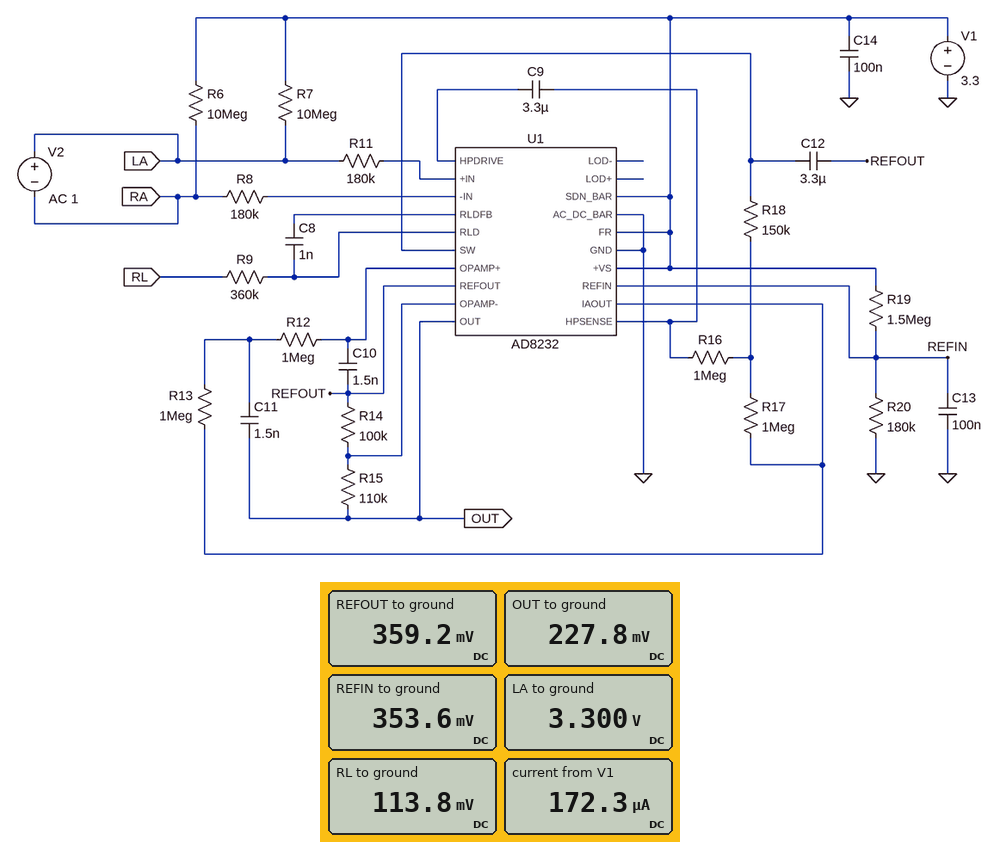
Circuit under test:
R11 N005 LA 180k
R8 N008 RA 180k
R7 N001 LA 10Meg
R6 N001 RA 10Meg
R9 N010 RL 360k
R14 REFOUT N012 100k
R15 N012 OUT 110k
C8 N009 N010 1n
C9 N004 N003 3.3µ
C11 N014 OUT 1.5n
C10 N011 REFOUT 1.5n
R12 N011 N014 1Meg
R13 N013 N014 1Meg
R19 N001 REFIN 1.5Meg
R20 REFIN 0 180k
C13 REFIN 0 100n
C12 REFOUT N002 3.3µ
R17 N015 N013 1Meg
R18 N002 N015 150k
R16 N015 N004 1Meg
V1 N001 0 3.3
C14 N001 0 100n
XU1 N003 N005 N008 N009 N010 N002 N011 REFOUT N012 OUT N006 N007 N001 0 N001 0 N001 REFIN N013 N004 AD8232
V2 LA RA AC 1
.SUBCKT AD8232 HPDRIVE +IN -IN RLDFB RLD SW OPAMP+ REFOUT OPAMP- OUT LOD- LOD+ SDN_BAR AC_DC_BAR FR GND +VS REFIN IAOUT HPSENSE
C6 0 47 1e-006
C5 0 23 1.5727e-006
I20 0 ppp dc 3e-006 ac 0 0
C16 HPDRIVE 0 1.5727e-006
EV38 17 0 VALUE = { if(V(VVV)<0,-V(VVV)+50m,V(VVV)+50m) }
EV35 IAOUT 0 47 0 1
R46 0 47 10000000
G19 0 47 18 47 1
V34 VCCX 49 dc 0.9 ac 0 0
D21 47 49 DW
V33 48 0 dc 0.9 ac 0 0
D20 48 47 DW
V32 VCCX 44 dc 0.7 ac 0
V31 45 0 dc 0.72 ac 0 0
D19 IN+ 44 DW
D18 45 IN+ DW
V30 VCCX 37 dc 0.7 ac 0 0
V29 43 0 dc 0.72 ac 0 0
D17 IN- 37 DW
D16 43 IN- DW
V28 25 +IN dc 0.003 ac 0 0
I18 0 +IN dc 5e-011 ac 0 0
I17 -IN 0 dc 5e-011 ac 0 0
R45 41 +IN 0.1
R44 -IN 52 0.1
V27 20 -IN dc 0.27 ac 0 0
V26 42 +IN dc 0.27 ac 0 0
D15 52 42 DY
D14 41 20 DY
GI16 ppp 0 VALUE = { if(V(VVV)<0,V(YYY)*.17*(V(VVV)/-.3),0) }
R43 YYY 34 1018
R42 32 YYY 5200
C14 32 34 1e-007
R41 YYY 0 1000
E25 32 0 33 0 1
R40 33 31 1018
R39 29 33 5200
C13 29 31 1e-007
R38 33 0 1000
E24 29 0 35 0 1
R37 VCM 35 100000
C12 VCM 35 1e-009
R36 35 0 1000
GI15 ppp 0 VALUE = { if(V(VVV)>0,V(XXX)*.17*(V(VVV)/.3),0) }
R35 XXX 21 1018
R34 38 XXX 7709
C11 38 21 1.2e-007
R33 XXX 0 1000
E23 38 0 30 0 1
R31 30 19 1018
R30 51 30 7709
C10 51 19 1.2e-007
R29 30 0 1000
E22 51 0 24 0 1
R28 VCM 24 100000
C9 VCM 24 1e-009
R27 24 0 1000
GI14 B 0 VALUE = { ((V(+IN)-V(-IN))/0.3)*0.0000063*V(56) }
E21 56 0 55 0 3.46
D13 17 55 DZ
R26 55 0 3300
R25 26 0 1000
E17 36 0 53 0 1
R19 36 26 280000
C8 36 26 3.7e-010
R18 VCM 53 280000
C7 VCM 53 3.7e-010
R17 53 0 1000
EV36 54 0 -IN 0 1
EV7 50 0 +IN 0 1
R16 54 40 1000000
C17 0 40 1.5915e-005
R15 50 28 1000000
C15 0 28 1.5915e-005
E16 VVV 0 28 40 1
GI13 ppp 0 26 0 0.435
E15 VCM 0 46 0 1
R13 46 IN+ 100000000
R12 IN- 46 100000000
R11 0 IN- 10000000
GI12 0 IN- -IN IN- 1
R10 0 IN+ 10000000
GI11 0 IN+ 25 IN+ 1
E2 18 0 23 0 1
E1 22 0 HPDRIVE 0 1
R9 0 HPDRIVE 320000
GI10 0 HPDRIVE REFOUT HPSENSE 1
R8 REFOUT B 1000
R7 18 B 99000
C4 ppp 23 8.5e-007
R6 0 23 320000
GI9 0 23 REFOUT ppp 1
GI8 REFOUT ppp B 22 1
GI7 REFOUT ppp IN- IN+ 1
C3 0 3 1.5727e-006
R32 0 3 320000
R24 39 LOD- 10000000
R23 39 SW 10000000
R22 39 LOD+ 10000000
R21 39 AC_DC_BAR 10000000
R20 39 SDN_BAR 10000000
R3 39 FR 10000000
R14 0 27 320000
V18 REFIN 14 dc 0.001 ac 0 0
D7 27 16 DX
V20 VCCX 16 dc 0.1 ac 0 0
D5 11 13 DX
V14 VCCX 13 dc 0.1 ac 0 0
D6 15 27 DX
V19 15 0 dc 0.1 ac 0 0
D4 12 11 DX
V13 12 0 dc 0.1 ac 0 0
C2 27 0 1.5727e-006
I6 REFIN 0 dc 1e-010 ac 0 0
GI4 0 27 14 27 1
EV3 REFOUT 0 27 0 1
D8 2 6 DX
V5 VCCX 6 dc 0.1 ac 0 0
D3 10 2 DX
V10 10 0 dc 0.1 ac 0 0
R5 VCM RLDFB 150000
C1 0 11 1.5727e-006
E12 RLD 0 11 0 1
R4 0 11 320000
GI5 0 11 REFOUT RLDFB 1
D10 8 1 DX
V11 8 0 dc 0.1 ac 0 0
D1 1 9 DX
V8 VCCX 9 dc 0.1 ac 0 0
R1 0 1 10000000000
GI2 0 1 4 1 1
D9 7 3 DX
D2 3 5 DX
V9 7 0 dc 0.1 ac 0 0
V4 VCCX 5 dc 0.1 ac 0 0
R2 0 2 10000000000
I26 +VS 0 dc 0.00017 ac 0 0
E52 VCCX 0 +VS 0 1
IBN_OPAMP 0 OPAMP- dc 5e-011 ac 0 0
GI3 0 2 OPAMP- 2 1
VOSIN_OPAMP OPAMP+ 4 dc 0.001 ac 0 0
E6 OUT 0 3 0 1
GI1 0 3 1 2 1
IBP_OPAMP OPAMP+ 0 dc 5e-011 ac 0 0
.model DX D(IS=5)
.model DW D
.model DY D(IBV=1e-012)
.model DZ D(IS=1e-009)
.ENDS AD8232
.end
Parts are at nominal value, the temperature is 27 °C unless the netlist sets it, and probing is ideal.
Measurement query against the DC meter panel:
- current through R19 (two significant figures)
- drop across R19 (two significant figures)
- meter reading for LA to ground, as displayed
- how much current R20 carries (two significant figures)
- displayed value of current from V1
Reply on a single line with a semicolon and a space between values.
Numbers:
2.0 µA; 2.9 V; 3.300 V; 2.0 µA; 172.3 µA
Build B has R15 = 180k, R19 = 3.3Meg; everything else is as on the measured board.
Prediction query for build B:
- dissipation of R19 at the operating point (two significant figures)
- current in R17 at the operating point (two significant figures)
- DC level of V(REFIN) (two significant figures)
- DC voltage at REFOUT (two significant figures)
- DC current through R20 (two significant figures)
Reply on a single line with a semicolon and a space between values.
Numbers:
3.0 µW; 150 nA; 170 mV; 230 mV; 950 nA
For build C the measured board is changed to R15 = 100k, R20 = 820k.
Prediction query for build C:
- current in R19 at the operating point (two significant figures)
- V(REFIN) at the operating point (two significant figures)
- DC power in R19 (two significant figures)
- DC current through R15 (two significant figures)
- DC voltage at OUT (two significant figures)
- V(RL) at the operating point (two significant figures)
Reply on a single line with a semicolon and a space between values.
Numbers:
1.4 µA; 1.2 V; 3.0 µW; 780 nA; 1.0 V; 120 mV
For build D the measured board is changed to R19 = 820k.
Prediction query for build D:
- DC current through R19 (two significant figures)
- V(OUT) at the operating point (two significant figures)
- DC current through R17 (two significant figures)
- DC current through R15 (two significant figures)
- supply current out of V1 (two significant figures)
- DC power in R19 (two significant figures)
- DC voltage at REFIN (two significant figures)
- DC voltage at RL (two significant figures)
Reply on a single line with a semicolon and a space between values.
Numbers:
3.3 µA; 360 mV; 120 nA; 1.1 µA; 170 µA; 8.9 µW; 590 mV; 120 mV
